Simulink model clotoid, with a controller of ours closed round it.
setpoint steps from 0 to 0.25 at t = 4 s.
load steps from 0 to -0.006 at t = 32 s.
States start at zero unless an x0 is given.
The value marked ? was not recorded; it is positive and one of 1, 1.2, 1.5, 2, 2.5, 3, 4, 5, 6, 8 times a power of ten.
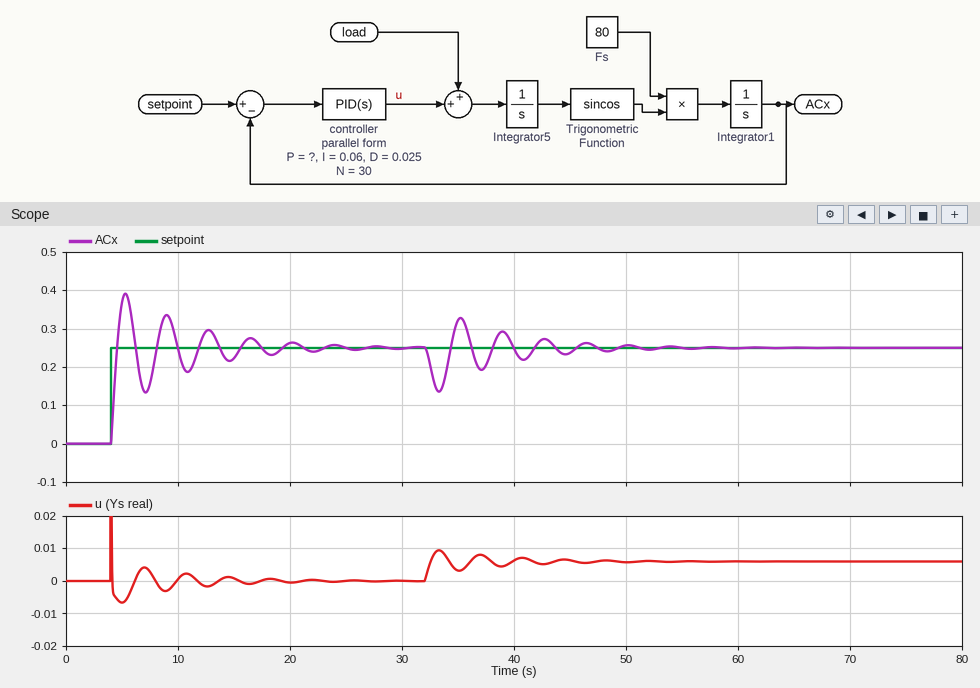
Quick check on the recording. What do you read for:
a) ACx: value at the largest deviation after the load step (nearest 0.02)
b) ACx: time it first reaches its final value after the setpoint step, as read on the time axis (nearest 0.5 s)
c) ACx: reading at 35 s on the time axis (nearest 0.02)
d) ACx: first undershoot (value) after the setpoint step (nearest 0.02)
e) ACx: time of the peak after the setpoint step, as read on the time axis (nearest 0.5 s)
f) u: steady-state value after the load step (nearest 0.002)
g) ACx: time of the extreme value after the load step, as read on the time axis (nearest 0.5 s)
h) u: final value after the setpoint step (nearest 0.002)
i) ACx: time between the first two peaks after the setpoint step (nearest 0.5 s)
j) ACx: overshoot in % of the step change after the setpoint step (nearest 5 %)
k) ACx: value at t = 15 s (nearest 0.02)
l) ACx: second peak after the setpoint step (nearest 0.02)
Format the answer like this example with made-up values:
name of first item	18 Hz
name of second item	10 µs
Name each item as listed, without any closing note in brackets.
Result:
ACx: value at the largest deviation after the load step	0.14
ACx: time it first reaches its final value after the setpoint step, as read on the time axis	4.5 s
ACx: reading at 35 s on the time axis	0.32
ACx: first undershoot (value) after the setpoint step	0.14
ACx: time of the peak after the setpoint step, as read on the time axis	5.5 s
u: steady-state value after the load step	0.006
ACx: time of the extreme value after the load step, as read on the time axis	33.5 s
u: final value after the setpoint step	0.000
ACx: time between the first two peaks after the setpoint step	3.5 s
ACx: overshoot in % of the step change after the setpoint step	55 %
ACx: value at t = 15 s	0.22
ACx: second peak after the setpoint step	0.34
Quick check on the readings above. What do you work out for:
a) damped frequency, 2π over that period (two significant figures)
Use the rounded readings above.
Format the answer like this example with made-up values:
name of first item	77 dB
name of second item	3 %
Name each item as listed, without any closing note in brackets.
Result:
damped frequency, 2π over that period	1.8 rad/s
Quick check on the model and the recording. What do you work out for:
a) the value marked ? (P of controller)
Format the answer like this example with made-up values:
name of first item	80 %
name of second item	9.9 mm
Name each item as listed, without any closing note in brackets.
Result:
the value marked ?	0.04
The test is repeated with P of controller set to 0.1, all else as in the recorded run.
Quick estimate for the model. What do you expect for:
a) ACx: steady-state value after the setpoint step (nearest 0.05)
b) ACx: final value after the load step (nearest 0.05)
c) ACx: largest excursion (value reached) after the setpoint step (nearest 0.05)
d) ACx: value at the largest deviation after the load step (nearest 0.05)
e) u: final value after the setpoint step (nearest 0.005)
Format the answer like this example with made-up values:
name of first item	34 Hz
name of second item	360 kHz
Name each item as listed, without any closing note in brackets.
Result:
ACx: steady-state value after the setpoint step	0.25
ACx: final value after the load step	0.25
ACx: largest excursion (value reached) after the setpoint step	0.40
ACx: value at the largest deviation after the load step	0.20
u: final value after the setpoint step	0.000
